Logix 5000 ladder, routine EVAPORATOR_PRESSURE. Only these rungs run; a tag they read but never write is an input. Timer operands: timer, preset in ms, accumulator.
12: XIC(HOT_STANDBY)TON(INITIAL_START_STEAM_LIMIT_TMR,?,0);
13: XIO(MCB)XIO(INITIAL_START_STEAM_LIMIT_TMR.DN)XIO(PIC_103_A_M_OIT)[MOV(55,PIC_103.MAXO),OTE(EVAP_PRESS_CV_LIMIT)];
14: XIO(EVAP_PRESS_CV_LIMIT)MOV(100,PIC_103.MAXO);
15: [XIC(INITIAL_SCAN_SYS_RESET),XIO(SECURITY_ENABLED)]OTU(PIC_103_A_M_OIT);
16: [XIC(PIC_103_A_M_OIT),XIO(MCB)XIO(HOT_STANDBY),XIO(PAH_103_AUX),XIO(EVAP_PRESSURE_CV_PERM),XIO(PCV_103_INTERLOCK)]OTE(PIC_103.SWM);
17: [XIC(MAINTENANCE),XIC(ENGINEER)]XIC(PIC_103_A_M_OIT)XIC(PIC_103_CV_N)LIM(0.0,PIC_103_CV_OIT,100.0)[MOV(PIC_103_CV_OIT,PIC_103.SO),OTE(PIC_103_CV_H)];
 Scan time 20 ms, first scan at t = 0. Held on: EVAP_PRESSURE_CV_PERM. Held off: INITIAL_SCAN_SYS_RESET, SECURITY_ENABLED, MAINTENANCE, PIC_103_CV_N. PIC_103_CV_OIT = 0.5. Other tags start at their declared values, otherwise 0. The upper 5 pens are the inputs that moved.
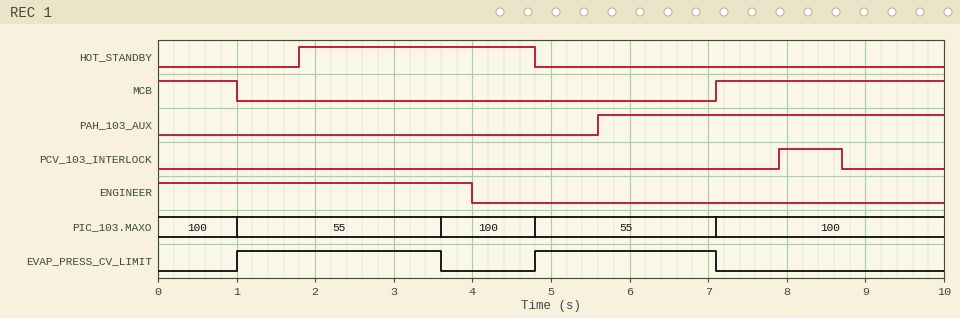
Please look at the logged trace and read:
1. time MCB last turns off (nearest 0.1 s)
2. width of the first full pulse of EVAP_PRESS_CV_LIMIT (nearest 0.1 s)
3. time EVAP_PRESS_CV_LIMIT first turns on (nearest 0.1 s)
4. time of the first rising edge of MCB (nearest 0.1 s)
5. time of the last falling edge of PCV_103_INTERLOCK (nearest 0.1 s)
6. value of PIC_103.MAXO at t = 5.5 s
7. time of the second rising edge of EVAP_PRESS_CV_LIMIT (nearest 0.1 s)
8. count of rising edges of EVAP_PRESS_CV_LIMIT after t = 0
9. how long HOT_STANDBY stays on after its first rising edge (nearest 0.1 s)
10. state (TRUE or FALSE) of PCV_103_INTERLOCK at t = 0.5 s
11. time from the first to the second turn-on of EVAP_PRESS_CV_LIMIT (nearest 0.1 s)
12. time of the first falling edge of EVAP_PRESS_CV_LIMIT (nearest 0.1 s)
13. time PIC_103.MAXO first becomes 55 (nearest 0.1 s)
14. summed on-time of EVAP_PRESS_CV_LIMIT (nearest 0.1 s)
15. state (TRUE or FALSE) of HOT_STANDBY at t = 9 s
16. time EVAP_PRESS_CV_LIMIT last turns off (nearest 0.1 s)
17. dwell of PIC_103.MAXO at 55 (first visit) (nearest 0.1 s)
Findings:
1.0 s
2.6 s
1.0 s
7.1 s
8.7 s
55
4.8 s
2
3.0 s
FALSE
3.8 s
3.6 s
1.0 s
4.9 s
FALSE
7.1 s
2.6 s
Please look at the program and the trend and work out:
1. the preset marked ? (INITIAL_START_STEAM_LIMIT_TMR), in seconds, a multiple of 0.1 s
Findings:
1.8 s
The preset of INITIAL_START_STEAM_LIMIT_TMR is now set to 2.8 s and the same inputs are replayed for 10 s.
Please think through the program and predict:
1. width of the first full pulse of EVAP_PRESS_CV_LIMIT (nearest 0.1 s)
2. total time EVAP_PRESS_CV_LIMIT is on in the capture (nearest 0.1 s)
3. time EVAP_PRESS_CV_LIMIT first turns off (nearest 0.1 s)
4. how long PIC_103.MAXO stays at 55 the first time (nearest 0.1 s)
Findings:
3.6 s
5.9 s
4.6 s
3.6 s
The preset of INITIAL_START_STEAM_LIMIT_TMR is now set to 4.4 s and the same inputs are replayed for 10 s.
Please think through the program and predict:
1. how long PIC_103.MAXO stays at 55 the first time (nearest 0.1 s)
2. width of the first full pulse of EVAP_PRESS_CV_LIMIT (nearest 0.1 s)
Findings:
6.1 s
6.1 s
